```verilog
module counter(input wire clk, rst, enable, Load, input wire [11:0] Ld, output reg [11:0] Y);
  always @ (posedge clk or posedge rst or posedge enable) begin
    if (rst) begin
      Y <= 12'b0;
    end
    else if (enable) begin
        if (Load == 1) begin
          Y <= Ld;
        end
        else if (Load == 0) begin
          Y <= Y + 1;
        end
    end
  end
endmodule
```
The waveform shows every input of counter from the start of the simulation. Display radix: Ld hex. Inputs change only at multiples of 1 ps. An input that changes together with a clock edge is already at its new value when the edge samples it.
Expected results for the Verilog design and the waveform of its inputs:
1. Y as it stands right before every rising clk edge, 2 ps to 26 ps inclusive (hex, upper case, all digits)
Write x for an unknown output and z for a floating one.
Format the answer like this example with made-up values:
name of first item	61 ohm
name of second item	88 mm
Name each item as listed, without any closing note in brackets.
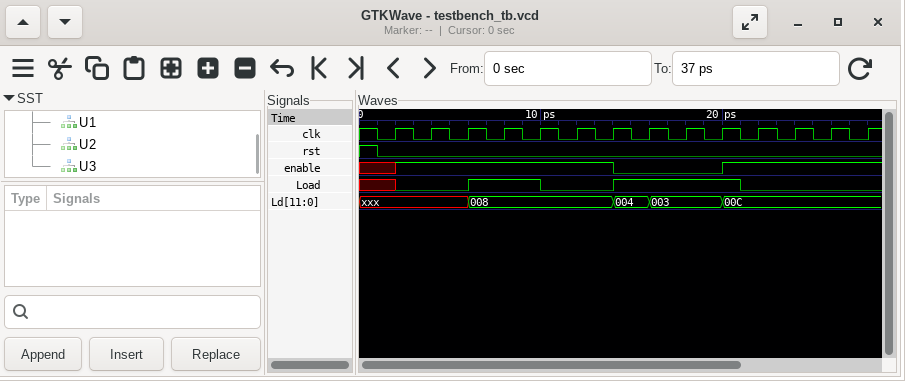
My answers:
Y as it stands right before every rising clk edge, 2 ps to 26 ps inclusive	000, 002, 003, 008, 008, 009, 00A, 00A, 00A, 00A, 00C, 00D, 00E
